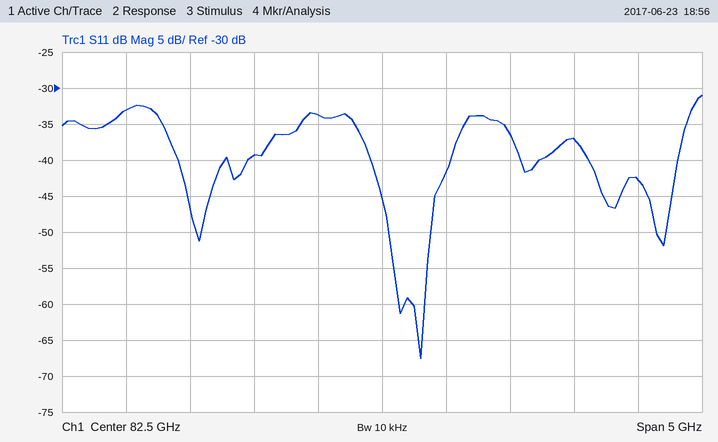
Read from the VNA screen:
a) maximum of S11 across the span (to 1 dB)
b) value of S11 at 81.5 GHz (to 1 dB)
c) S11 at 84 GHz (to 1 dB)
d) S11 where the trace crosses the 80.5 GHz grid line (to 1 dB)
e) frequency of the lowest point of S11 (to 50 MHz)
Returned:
-31 dB
-39 dB
-37 dB
-33 dB
82.80 GHz
